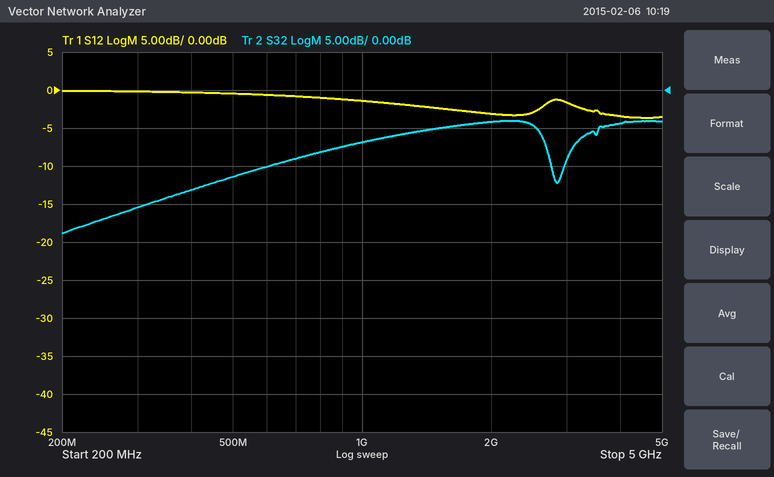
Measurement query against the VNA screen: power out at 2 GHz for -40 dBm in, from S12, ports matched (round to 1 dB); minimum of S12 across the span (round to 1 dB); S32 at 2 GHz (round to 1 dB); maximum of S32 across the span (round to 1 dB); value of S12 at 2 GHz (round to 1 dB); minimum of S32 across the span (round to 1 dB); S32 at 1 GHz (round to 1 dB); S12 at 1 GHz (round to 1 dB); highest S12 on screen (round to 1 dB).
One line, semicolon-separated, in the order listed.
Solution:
-43 dBm; -4 dB; -4 dB; -4 dB; -3 dB; -19 dB; -7 dB; -1 dB; 0 dB
